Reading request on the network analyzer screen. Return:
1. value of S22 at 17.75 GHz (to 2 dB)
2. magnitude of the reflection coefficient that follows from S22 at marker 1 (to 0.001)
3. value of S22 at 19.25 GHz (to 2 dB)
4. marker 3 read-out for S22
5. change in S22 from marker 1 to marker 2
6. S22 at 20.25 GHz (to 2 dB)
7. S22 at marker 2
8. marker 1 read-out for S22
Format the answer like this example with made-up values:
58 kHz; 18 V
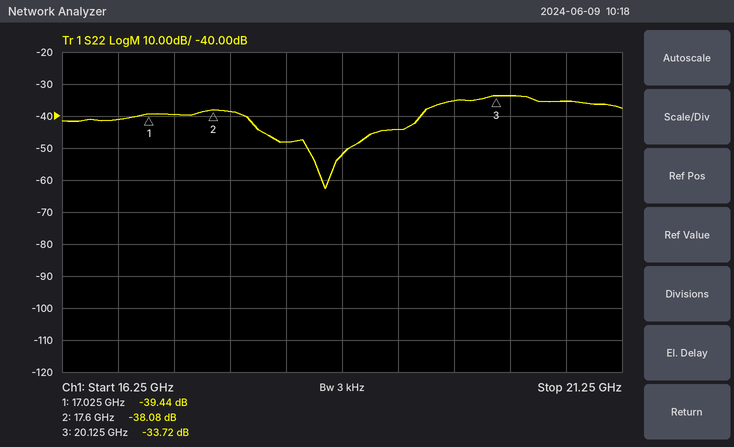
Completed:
-38 dB; 0.011; -44 dB; -33.72 dB; 1.36 dB; -34 dB; -38.08 dB; -39.44 dB
